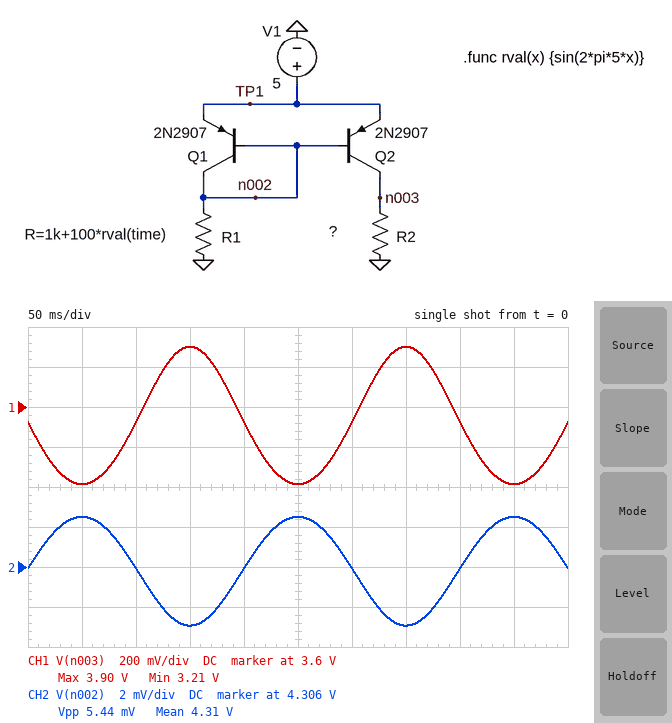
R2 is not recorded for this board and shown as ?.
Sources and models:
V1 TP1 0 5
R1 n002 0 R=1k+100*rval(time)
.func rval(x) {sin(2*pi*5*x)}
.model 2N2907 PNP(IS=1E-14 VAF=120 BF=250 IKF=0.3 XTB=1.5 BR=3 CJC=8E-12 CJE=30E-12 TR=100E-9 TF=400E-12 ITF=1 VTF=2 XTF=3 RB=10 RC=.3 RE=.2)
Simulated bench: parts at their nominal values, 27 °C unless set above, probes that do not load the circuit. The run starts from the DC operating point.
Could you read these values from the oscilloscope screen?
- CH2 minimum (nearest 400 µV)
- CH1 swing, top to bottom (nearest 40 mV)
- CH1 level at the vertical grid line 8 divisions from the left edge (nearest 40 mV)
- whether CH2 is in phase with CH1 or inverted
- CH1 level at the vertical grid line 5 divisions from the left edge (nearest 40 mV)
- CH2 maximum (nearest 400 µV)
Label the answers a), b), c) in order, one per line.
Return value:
a) 4.3032 V
b) 680 mV
c) 3.52 V
d) inverted
e) 3.20 V
f) 4.3084 V
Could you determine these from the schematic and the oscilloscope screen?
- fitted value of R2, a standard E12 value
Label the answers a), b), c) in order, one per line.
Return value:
a) 820 Ω
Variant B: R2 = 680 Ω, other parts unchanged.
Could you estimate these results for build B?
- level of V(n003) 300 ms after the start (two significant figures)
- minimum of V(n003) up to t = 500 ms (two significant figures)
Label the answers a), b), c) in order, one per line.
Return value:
a) 2.9 V
b) 2.7 V
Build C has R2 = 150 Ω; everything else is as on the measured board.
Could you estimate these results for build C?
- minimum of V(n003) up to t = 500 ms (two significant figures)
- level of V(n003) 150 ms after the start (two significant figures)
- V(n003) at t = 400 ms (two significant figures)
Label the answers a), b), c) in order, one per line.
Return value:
a) 600 mV
b) 730 mV
c) 660 mV
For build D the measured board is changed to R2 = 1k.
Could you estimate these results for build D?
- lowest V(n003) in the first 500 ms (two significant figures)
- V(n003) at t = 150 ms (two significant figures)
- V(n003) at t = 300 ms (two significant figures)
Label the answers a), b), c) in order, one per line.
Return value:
a) 3.9 V
b) 4.7 V
c) 4.3 V
